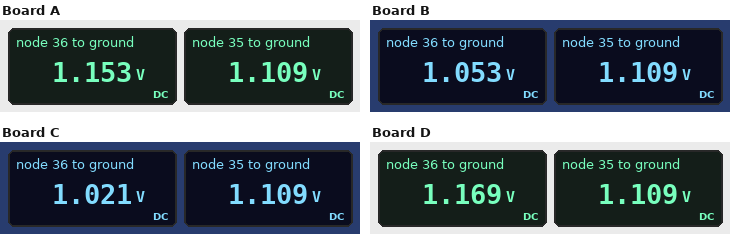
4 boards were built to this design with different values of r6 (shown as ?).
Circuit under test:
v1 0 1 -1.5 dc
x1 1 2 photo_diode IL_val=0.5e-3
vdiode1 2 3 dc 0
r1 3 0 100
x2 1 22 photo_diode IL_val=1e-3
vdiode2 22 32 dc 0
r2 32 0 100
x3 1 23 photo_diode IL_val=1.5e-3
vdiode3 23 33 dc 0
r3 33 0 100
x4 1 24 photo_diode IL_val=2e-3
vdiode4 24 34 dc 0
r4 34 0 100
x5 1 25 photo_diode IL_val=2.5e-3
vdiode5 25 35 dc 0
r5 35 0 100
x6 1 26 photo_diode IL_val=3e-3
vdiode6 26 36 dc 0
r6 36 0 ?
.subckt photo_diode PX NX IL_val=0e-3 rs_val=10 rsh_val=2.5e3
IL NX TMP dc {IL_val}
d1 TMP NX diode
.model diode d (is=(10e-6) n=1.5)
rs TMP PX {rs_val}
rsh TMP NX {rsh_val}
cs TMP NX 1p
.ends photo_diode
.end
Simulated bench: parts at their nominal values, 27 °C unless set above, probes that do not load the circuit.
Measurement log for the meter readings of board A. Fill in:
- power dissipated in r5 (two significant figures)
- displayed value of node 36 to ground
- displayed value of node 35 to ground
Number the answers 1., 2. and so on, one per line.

1. 12 mW
2. 1.153 V
3. 1.109 V
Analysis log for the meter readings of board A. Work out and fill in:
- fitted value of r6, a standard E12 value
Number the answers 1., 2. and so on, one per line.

1. 150 Ω
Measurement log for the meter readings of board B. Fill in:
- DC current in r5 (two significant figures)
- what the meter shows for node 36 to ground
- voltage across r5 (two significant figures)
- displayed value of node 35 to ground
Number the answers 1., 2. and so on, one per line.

1. 11 mA
2. 1.053 V
3. 1.1 V
4. 1.109 V
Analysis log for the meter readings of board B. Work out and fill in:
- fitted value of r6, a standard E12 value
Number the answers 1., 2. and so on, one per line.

1. 68 Ω
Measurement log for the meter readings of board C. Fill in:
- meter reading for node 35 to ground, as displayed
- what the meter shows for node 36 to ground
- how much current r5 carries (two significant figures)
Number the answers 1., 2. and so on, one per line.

1. 1.109 V
2. 1.021 V
3. 11 mA
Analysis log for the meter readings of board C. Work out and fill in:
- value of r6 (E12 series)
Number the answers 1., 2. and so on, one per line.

1. 56 Ω
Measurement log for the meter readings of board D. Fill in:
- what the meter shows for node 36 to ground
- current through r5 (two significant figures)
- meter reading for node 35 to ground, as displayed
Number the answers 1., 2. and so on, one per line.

1. 1.169 V
2. 11 mA
3. 1.109 V
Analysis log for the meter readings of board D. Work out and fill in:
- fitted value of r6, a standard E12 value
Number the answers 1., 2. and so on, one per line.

1. 180 Ω
